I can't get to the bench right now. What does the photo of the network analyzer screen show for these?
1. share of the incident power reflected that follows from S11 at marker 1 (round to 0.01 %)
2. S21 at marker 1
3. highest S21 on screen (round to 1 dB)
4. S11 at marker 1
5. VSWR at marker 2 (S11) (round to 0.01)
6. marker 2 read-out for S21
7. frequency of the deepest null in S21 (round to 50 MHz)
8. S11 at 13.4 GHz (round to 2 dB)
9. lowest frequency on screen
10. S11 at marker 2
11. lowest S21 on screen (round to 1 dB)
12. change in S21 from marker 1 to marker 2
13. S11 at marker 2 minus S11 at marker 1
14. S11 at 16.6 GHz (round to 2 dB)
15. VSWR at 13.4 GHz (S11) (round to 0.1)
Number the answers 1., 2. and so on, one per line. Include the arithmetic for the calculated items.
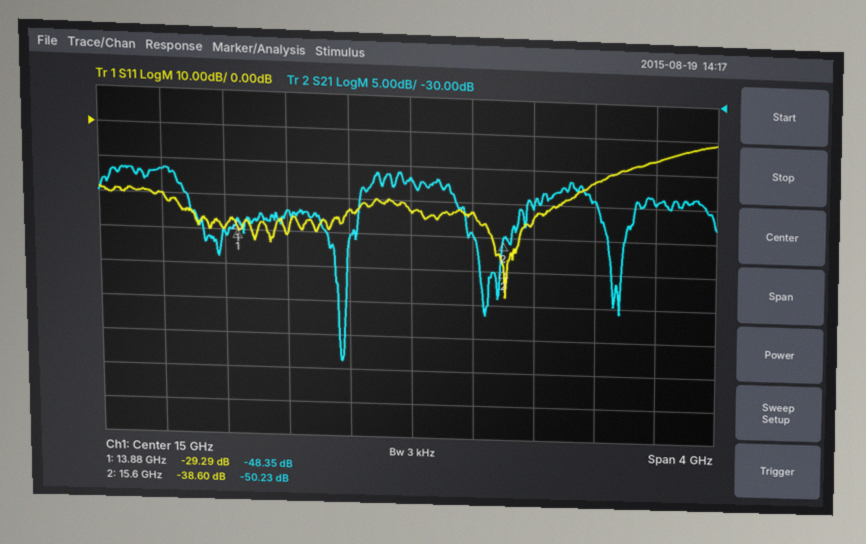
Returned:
1. 10^(-29.29/10) ≈ 0.12 %
2. -48.35 dB
3. -41 dB
4. -29.29 dB
5. (1 + 0.0117)/(1 − 0.0117) ≈ 1.02
6. -50.23 dB
7. 14.55 GHz
8. -20 dB
9. 13 GHz
10. -38.60 dB
11. -69 dB
12. -50.23 − (-48.35) = -1.88 dB
13. -38.6 − (-29.29) = -9.31 dB
14. -6 dB
15. |Γ| = 10^(-20/20) = 0.1000; VSWR = (1 + 0.1000)/(1 − 0.1000) ≈ 1.2
